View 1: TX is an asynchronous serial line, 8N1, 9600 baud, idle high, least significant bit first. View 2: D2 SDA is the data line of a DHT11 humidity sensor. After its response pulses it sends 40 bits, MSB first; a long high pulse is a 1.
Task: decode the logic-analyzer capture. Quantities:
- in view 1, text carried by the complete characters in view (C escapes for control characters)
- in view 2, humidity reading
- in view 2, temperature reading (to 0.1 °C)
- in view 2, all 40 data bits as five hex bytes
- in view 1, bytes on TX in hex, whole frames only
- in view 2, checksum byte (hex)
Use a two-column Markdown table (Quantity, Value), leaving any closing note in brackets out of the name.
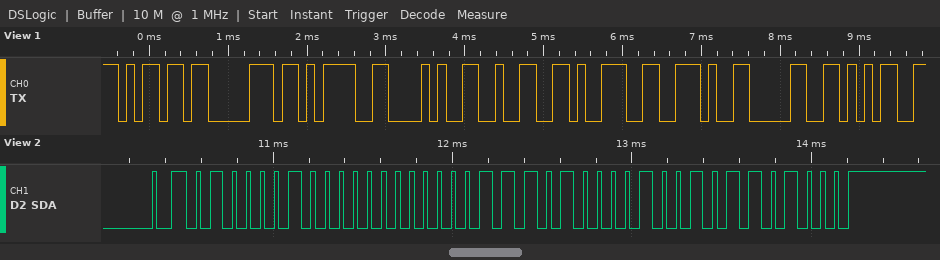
| Quantity | Value |
|---|---|
| in view 1, text carried by the complete characters in view | "mp=(29.05" |
| in view 2, humidity reading | 66 % |
| in view 2, temperature reading | 29.9 °C |
| in view 2, all 40 data bits as five hex bytes | 42 00 1D 09 68 |
| in view 1, bytes on TX in hex, whole frames only | 0x6D 0x70 0x3D 0x28 0x32 0x39 0x2E 0x30 0x35 |
| in view 2, checksum byte | 0x68 |
